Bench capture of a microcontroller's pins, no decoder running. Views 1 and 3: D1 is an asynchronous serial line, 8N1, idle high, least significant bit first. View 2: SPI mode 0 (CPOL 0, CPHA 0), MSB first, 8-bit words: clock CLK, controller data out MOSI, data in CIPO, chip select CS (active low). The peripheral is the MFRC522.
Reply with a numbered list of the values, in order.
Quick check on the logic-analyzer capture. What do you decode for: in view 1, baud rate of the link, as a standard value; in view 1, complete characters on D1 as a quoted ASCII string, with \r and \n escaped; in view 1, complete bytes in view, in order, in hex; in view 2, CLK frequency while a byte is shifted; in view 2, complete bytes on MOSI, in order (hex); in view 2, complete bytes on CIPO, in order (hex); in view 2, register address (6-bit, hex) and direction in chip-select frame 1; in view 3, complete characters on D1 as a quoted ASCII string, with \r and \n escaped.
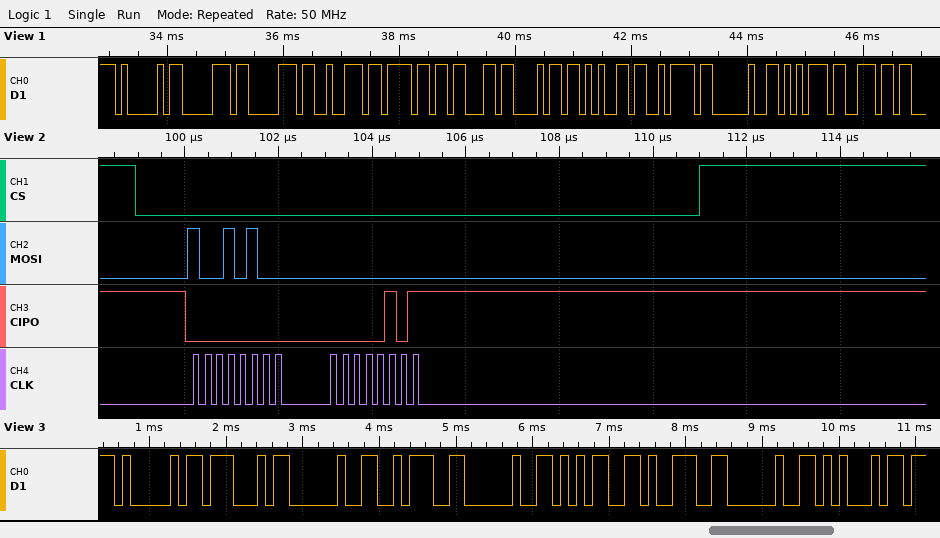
1. 9600 baud
2. "Approchez un"
3. 41 70 70 72 6F 63 68 65 7A 20 75 6E
4. 4 MHz
5. 94 00
6. 00 05
7. 0x0A read
8. "AG : 59 E"
